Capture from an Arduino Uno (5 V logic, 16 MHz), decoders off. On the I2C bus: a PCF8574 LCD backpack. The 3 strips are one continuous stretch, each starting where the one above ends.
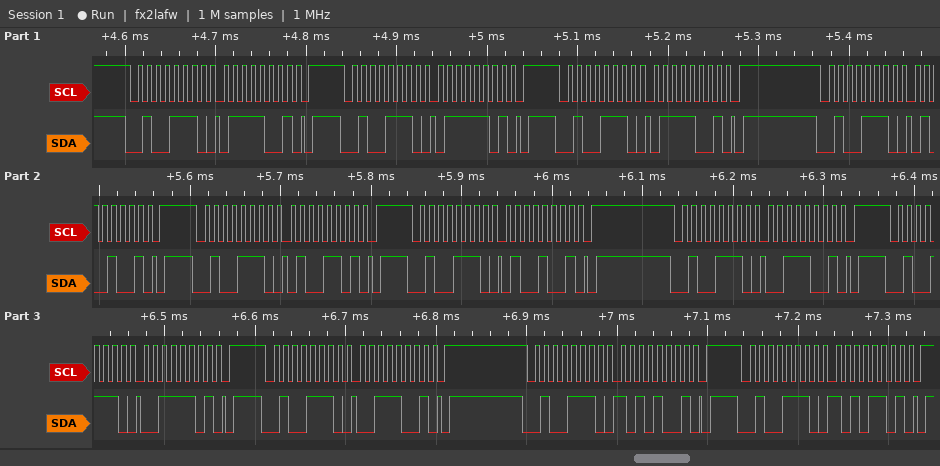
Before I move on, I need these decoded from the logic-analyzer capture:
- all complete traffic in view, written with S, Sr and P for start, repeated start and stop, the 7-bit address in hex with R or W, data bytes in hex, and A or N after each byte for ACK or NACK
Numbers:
S 27W A 79 A P S 27W A 7D A P S 27W A 79 A P S 27W A 49 A P S 27W A 4D A P S 27W A 49 A P S 27W A 39 A P S 27W A 3D A P S 27W A 39 A P S 27W A A9 A P S 27W A AD A P
